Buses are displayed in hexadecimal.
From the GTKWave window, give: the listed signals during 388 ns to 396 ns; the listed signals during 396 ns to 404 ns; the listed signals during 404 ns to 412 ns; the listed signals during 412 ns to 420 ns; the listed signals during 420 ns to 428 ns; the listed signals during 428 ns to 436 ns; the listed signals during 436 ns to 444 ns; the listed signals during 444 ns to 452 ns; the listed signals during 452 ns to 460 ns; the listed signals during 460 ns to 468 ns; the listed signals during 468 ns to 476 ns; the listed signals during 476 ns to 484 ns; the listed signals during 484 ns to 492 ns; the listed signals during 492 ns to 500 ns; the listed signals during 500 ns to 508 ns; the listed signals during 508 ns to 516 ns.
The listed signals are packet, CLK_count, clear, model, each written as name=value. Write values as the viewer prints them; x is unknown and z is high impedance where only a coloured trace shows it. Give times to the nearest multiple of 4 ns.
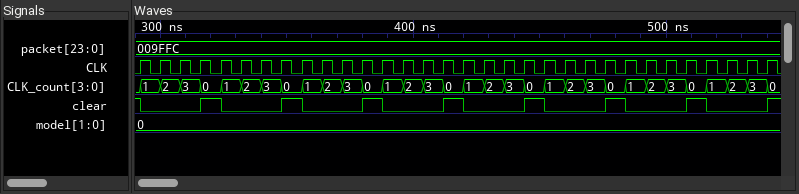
packet=009FFC, CLK_count=1, clear=0, model=0
packet=009FFC, CLK_count=2, clear=0, model=0
packet=009FFC, CLK_count=3, clear=0, model=0
packet=009FFC, CLK_count=0, clear=1, model=0
packet=009FFC, CLK_count=1, clear=0, model=0
packet=009FFC, CLK_count=2, clear=0, model=0
packet=009FFC, CLK_count=3, clear=0, model=0
packet=009FFC, CLK_count=0, clear=1, model=0
packet=009FFC, CLK_count=1, clear=0, model=0
packet=009FFC, CLK_count=2, clear=0, model=0
packet=009FFC, CLK_count=3, clear=0, model=0
packet=009FFC, CLK_count=0, clear=1, model=0
packet=009FFC, CLK_count=1, clear=0, model=0
packet=009FFC, CLK_count=2, clear=0, model=0
packet=009FFC, CLK_count=3, clear=0, model=0
packet=009FFC, CLK_count=0, clear=1, model=0
